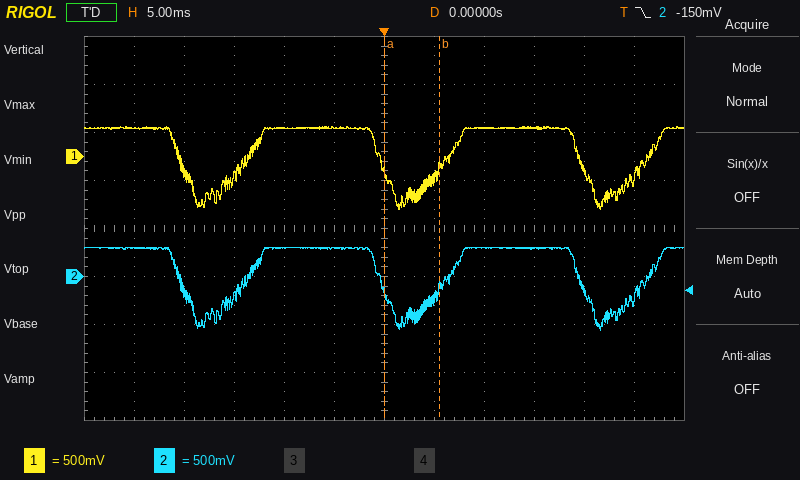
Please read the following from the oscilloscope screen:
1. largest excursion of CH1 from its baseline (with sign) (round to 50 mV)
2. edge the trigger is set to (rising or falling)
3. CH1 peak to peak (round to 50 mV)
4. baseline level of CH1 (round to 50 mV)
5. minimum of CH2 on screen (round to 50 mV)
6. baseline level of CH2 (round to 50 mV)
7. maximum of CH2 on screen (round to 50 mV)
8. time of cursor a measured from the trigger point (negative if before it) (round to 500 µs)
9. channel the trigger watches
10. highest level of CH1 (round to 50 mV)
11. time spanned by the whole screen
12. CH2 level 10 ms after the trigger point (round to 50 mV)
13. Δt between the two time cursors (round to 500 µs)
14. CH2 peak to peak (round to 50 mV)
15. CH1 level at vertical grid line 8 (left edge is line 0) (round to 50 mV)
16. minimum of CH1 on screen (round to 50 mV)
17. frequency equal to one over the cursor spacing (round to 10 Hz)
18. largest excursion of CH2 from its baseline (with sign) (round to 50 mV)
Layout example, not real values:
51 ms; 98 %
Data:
-850 mV; falling; 850 mV; 300 mV; -550 mV; 300 mV; 300 mV; 0.0 ms; CH2; 300 mV; 60 ms; 300 mV; 5.5 ms; 850 mV; 300 mV; -550 mV; 180 Hz; -850 mV
